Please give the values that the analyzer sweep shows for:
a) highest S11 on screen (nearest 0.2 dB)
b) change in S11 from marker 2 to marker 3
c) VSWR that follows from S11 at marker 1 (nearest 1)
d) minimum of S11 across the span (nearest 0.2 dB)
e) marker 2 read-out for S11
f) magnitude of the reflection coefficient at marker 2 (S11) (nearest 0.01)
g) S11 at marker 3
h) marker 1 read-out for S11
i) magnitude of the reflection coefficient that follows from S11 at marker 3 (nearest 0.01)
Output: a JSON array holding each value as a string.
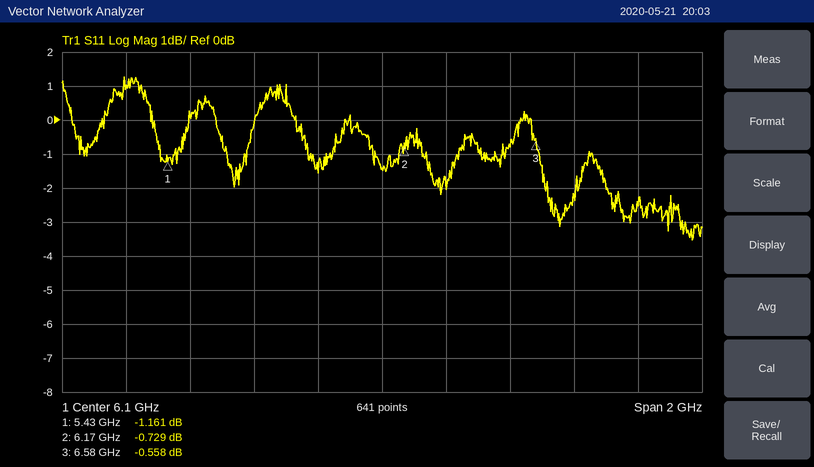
["1.2 dB", "0.171 dB", "15", "-3.6 dB", "-0.729 dB", "0.92", "-0.558 dB", "-1.161 dB", "0.94"]
